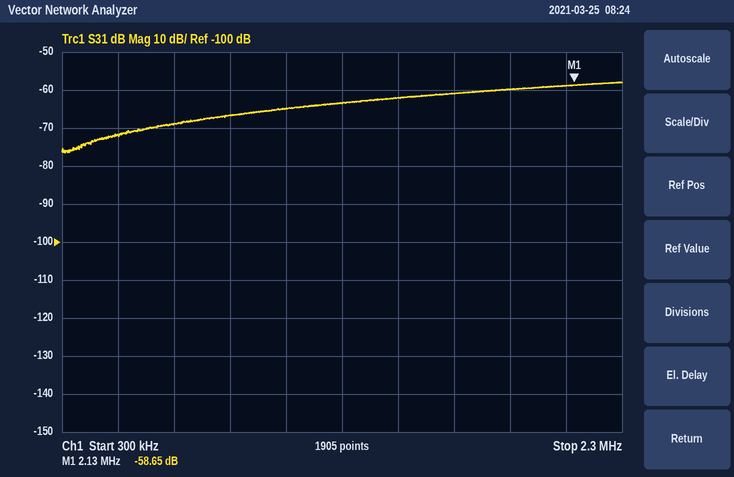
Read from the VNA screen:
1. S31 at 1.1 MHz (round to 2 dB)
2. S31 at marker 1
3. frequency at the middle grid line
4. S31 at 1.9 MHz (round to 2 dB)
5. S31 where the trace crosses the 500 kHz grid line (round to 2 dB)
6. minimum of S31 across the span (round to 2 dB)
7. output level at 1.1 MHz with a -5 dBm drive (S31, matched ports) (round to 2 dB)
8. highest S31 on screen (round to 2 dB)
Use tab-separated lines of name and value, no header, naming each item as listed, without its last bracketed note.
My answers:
S31 at 1.1 MHz	-64 dB
S31 at marker 1	-58.65 dB
frequency at the middle grid line	1.3 MHz
S31 at 1.9 MHz	-60 dB
S31 where the trace crosses the 500 kHz grid line	-72 dB
minimum of S31 across the span	-76 dB
output level at 1.1 MHz with a -5 dBm drive (S31, matched ports)	-70 dBm
highest S31 on screen	-58 dB
